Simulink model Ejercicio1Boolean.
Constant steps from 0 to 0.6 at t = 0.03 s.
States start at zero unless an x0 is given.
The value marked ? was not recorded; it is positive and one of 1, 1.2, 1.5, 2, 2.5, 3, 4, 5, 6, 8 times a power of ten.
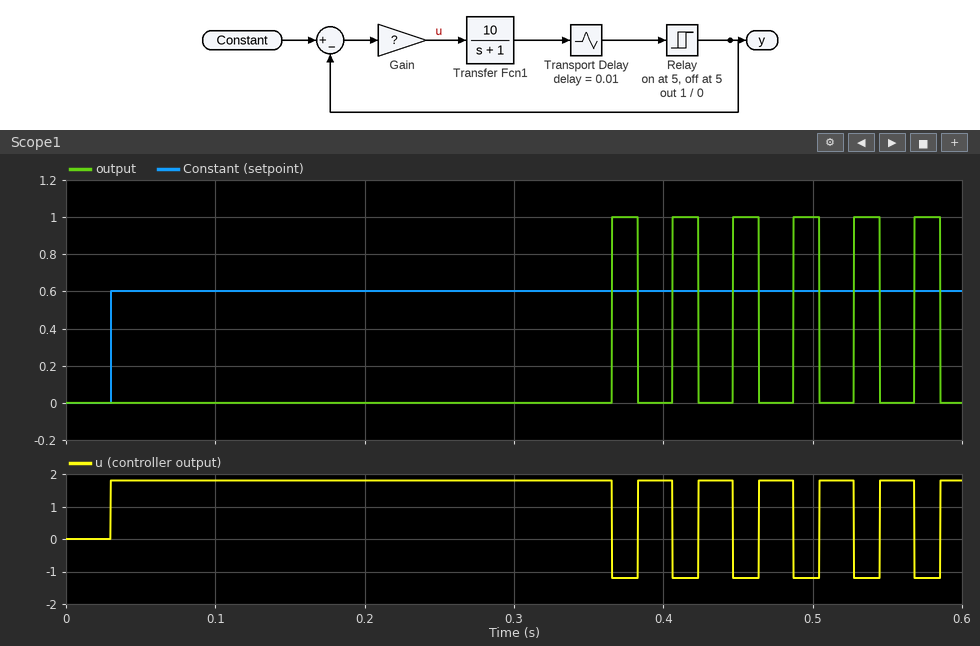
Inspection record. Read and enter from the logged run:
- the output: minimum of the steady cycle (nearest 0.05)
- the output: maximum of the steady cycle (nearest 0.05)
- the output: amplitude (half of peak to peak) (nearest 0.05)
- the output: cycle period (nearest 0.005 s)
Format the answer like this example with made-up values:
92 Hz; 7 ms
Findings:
0.00; 1.00; 0.50; 0.040 s
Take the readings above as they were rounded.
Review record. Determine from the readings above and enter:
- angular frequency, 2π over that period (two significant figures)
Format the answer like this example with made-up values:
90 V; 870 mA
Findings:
160 rad/s
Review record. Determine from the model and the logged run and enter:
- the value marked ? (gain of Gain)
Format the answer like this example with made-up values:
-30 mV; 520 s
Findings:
3
